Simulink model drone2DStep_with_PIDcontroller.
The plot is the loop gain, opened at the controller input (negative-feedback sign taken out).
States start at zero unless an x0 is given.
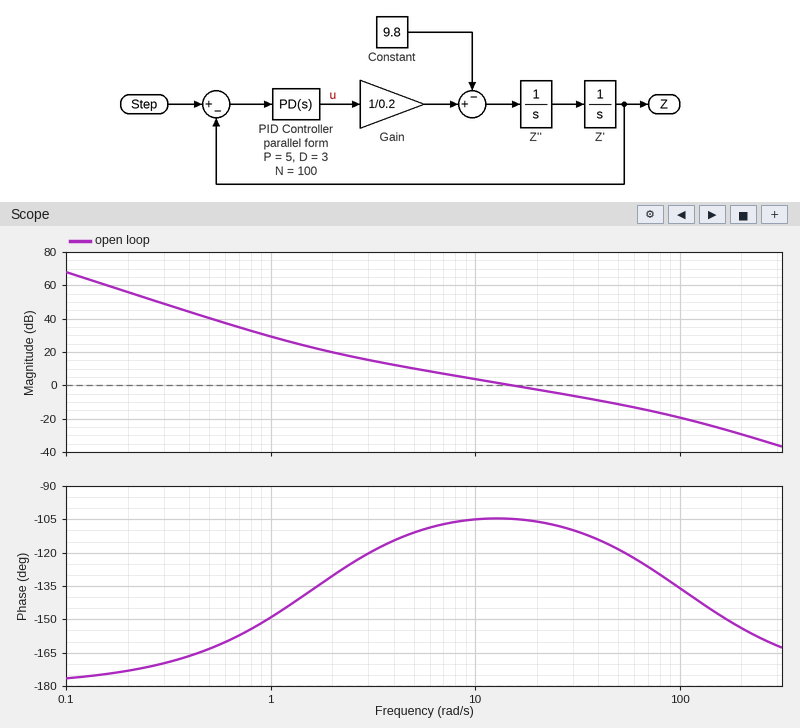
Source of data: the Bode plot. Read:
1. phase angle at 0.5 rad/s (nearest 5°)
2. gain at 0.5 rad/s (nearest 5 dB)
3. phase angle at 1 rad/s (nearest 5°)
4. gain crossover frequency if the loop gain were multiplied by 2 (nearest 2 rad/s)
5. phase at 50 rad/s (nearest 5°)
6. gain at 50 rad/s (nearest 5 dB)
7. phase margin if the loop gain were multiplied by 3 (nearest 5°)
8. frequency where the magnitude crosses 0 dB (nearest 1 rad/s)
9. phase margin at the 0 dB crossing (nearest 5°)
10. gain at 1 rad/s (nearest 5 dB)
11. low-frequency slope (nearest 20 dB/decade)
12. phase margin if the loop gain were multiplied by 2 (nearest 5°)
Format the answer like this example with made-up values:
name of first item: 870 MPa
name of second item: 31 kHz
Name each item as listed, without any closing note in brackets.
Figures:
phase angle at 0.5 rad/s: -165°
gain at 0.5 rad/s: 40 dB
phase angle at 1 rad/s: -150°
gain crossover frequency if the loop gain were multiplied by 2: 30 rad/s
phase at 50 rad/s: -120°
gain at 50 rad/s: -10 dB
phase margin if the loop gain were multiplied by 3: 65°
frequency where the magnitude crosses 0 dB: 15 rad/s
phase margin at the 0 dB crossing: 75°
gain at 1 rad/s: 30 dB
low-frequency slope: -40 dB/decade
phase margin if the loop gain were multiplied by 2: 70°
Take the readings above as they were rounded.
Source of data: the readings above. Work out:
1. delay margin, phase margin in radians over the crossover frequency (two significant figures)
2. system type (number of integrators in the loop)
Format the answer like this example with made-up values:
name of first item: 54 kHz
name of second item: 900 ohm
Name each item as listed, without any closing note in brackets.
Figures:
delay margin, phase margin in radians over the crossover frequency: 0.087 s
system type: 2
